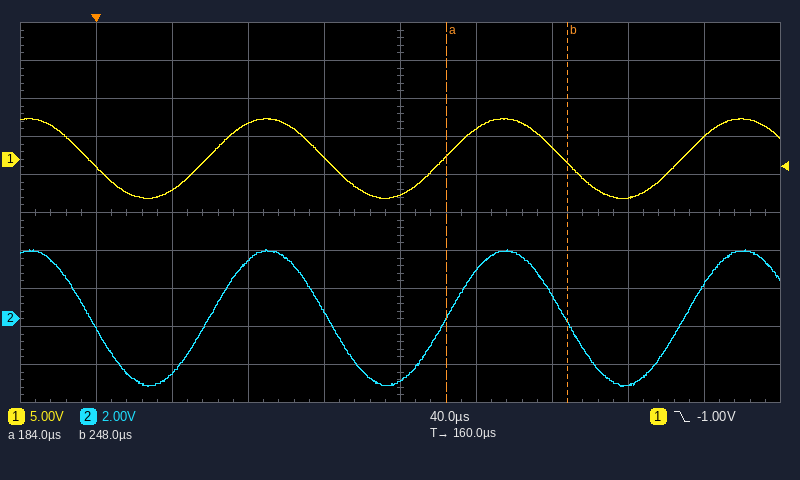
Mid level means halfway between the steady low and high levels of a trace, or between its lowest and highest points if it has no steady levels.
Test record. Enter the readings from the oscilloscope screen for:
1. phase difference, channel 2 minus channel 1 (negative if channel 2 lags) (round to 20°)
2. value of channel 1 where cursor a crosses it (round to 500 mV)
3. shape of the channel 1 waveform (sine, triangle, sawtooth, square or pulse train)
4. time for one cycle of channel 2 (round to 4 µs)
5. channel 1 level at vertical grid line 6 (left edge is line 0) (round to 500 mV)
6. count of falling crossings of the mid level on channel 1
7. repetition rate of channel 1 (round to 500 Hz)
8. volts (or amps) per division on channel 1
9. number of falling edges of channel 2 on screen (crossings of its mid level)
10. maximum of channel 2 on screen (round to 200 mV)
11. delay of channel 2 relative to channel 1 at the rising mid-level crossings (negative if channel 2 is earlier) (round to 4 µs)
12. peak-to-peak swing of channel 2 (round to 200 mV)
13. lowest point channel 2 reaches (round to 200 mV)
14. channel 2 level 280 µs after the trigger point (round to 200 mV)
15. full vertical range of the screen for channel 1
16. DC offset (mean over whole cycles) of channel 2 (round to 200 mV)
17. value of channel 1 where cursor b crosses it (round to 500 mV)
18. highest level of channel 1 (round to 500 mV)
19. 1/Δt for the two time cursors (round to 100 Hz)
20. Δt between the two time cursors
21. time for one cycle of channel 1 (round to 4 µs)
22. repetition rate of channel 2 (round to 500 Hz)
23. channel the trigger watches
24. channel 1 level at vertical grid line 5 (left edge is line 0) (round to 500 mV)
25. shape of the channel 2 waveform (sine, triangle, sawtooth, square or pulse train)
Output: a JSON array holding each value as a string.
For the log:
["0°", "500 mV", "sine", "124 µs", "4.0 V", "3", "8.0 kHz", "5 V", "3", "3.6 V", "0 µs", "7.2 V", "-3.6 V", "-3.4 V", "50 V", "0.0 V", "-500 mV", "5.5 V", "15.6 kHz", "64 µs", "124 µs", "8.0 kHz", "channel 1", "-4.5 V", "sine"]
